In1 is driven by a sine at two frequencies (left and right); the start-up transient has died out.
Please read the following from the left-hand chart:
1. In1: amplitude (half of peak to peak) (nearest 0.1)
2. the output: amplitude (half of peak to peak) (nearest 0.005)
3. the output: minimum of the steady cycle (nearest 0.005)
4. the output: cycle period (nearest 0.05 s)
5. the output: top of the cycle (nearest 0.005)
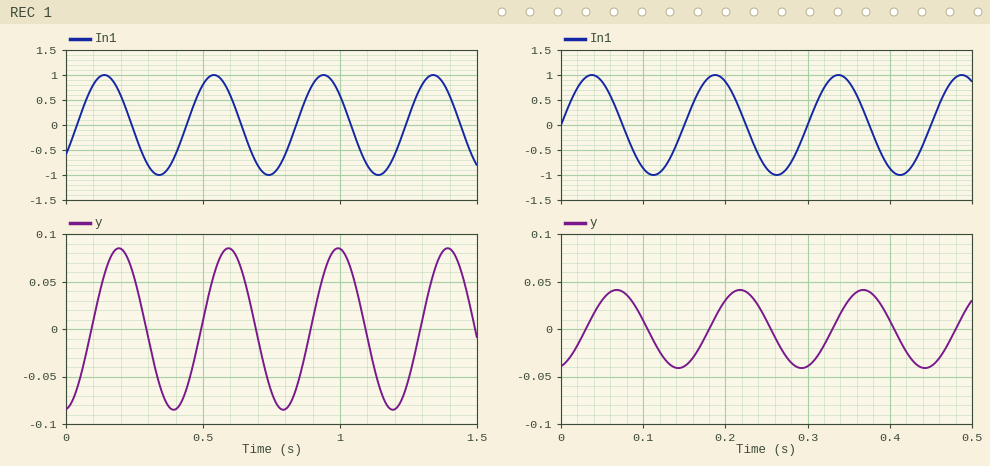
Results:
1.0
0.085
-0.085
0.40 s
0.085
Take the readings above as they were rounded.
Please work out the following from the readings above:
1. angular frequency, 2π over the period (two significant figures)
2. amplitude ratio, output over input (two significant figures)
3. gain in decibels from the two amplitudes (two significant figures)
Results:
16 rad/s
0.085
-21 dB
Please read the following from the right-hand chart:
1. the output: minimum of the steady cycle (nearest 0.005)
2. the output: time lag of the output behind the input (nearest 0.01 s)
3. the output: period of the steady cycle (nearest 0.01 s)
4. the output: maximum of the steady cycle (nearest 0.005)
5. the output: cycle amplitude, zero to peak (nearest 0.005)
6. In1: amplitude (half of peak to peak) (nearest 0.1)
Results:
-0.040
0.03 s
0.15 s
0.040
0.040
1.0
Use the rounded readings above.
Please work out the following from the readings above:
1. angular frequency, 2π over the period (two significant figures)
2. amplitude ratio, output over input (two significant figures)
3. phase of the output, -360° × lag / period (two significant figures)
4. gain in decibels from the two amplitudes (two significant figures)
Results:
42 rad/s
0.040
-72°
-28 dB
